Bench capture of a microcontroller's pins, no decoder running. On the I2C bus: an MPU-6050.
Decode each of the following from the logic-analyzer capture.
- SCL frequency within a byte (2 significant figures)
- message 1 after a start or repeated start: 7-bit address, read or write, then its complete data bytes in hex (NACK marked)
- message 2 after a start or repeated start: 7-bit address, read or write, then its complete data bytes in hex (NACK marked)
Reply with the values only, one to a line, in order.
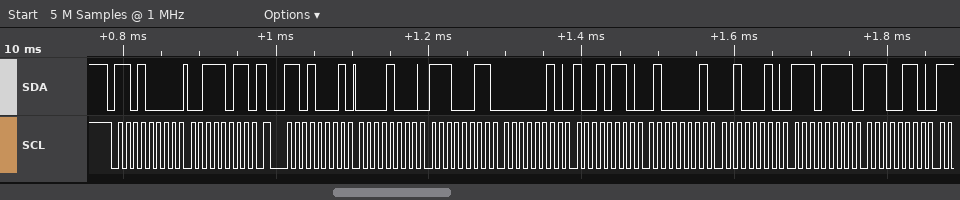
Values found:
100 kHz
0x68 write: 3B
0x68 read: 08 E3 02 96 41 22 EF E6
